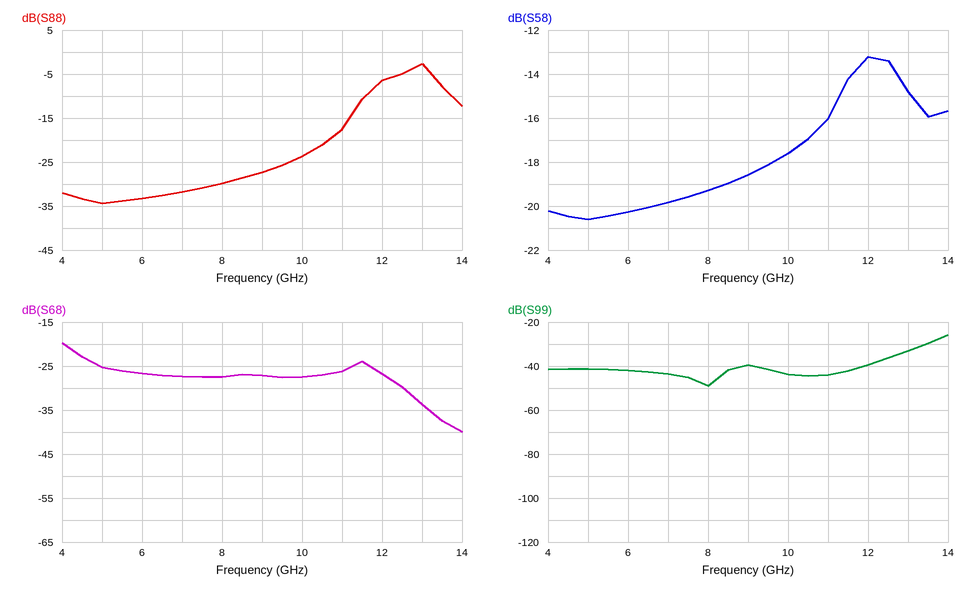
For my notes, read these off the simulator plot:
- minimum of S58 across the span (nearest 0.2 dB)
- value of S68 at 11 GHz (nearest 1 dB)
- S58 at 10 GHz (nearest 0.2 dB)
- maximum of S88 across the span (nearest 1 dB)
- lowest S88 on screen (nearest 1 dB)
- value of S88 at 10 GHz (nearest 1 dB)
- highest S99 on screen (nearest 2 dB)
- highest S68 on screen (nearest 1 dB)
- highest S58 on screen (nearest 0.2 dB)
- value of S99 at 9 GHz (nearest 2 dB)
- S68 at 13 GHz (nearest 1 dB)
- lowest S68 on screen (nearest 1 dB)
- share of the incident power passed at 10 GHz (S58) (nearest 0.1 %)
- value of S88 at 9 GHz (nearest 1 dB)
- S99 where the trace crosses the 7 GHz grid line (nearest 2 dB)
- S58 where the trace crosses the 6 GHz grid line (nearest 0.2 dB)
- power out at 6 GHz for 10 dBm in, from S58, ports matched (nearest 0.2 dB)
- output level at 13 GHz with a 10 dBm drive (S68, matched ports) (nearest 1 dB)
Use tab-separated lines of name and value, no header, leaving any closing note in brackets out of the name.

minimum of S58 across the span	-20.6 dB
value of S68 at 11 GHz	-26 dB
S58 at 10 GHz	-17.6 dB
maximum of S88 across the span	-3 dB
lowest S88 on screen	-34 dB
value of S88 at 10 GHz	-24 dB
highest S99 on screen	-26 dB
highest S68 on screen	-20 dB
highest S58 on screen	-13.2 dB
value of S99 at 9 GHz	-40 dB
S68 at 13 GHz	-34 dB
lowest S68 on screen	-40 dB
share of the incident power passed at 10 GHz (S58)	1.7 %
value of S88 at 9 GHz	-27 dB
S99 where the trace crosses the 7 GHz grid line	-44 dB
S58 where the trace crosses the 6 GHz grid line	-20.2 dB
power out at 6 GHz for 10 dBm in, from S58, ports matched	-10.2 dBm
output level at 13 GHz with a 10 dBm drive (S68, matched ports)	-24 dBm
